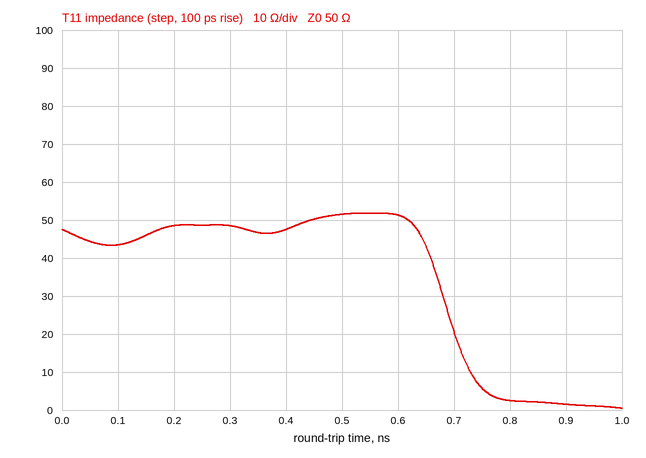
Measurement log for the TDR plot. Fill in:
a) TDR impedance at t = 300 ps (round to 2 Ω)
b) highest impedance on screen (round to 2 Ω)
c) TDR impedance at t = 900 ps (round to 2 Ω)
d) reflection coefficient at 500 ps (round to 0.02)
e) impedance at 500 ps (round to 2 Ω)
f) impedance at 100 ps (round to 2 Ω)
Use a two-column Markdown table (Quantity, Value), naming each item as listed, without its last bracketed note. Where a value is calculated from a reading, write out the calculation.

| Quantity | Value |
|---|---|
| TDR impedance at t = 300 ps | 48 Ω |
| highest impedance on screen | 52 Ω |
| TDR impedance at t = 900 ps | 2 Ω |
| reflection coefficient at 500 ps | (52 − 50)/(52 + 50) ≈ +0.02 |
| impedance at 500 ps | 52 Ω |
| impedance at 100 ps | 44 Ω |
